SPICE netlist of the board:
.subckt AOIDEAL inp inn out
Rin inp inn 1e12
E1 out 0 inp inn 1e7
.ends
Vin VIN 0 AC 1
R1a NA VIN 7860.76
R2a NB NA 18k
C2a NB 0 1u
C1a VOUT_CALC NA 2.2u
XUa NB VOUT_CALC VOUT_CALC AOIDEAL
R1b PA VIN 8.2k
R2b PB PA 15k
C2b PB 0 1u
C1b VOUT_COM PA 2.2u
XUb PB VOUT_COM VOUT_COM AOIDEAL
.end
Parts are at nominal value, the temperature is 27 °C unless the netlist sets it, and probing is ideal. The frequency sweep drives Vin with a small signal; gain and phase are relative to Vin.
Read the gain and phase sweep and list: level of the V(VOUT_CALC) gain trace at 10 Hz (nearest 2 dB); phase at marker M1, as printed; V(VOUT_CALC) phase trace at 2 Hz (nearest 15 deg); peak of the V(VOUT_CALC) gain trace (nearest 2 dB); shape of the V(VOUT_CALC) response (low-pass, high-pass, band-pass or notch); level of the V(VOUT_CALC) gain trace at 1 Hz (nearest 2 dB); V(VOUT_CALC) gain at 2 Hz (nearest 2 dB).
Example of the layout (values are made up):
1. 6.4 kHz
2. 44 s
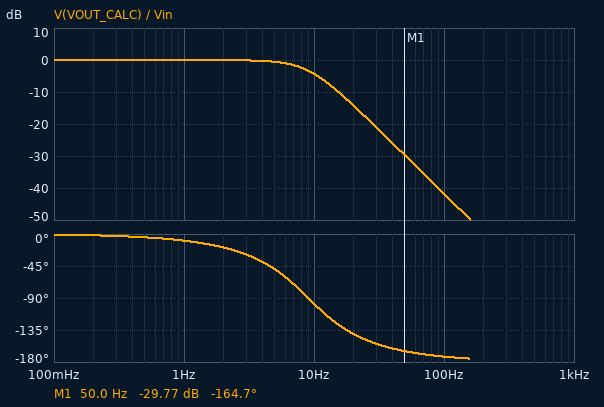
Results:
1. -4 dB
2. -164.7 deg
3. -15 deg
4. 0 dB
5. low-pass
6. 0 dB
7. 0 dB
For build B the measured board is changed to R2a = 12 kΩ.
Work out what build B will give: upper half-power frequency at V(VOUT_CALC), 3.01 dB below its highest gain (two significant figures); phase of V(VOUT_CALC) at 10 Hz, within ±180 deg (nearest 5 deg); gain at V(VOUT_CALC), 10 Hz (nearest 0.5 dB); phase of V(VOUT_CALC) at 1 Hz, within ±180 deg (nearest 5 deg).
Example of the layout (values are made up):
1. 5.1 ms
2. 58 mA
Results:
1. 11 Hz
2. -80 deg
3. -2.0 dB
4. -5 deg
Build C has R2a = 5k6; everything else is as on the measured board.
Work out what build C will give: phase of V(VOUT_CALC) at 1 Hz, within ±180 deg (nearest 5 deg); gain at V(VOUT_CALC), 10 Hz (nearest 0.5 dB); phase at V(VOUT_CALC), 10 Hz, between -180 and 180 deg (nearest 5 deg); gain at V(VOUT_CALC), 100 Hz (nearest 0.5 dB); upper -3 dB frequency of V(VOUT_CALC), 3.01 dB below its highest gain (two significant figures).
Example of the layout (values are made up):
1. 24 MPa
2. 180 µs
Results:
1. -5 deg
2. -0.5 dB
3. -55 deg
4. -31.5 dB
5. 17 Hz
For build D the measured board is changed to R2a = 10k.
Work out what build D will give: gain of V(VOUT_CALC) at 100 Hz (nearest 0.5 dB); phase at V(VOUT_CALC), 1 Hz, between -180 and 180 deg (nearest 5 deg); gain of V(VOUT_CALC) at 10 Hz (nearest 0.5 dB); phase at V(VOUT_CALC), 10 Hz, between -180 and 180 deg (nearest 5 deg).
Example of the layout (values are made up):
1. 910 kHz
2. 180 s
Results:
1. -36.5 dB
2. -5 deg
3. -1.5 dB
4. -75 deg
